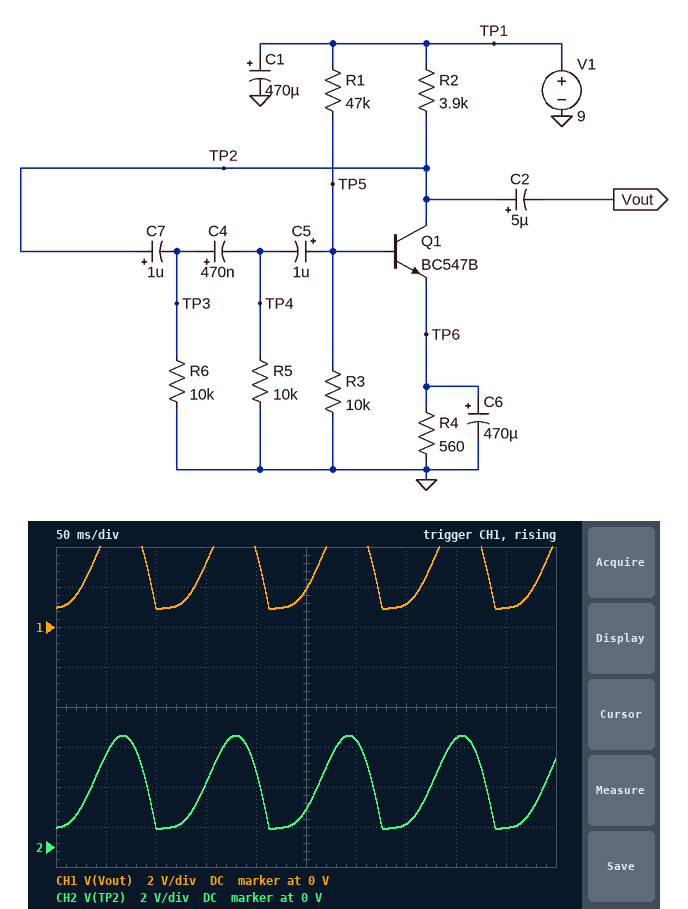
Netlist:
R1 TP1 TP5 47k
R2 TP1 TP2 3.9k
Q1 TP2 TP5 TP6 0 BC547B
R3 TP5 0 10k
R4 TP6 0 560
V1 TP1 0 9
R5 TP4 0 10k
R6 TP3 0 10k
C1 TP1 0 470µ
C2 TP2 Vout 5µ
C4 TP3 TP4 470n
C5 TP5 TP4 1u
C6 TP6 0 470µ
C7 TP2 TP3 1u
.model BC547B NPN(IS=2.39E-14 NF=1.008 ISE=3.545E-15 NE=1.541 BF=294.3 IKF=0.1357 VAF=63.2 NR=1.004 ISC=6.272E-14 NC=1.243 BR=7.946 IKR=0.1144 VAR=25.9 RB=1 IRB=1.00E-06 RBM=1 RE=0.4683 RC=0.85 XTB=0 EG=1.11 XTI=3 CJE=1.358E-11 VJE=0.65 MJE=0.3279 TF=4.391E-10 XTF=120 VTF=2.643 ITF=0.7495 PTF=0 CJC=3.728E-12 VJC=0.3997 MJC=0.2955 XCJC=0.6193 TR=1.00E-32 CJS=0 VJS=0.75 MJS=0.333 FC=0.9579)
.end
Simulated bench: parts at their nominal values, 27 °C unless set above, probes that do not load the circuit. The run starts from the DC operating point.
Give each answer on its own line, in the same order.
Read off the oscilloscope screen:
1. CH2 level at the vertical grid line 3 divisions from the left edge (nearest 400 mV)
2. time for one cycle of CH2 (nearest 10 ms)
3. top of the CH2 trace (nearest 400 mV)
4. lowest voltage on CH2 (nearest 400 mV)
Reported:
3.2 V
110 ms
5.6 V
800 mV
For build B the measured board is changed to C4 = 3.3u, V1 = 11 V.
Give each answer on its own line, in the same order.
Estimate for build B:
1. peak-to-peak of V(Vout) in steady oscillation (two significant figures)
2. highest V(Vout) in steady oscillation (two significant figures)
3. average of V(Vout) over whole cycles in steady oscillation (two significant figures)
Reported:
3.2 V
4.4 V
2.7 V
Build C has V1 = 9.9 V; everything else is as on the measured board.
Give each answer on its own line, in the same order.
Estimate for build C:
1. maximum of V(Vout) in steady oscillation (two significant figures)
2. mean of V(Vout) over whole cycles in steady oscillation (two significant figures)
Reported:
5.1 V
2.9 V
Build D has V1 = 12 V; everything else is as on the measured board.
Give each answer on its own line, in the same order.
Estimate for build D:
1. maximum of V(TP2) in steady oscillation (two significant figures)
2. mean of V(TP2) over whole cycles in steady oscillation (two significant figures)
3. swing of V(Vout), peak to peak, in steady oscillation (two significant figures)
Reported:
3.9 V
2.6 V
2.5 V
